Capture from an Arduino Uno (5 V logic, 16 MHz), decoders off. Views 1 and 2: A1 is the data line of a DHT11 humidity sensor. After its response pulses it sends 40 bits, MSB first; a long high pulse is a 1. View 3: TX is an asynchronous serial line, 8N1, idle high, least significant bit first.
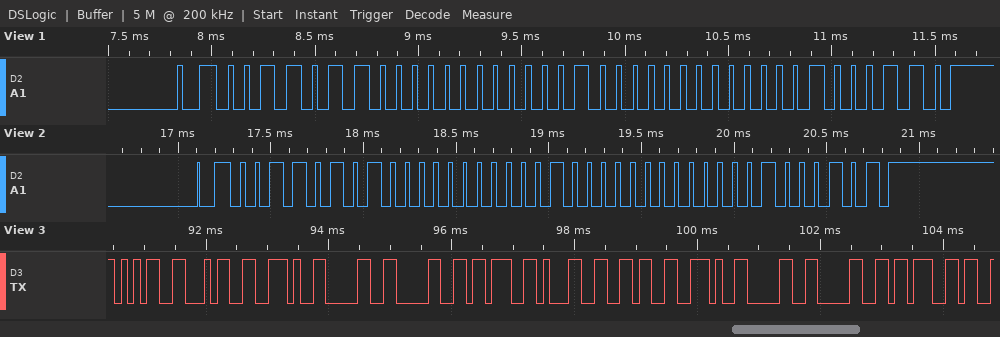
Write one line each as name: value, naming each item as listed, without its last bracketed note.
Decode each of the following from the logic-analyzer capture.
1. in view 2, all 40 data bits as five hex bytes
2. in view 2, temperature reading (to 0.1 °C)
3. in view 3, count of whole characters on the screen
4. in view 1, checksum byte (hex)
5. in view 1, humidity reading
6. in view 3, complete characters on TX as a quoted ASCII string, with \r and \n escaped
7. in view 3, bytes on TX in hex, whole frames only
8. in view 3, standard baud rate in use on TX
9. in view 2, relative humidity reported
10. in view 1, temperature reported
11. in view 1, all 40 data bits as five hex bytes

in view 2, all 40 data bits as five hex bytes: 35 00 10 00 45
in view 2, temperature reading: 16.0 °C
in view 3, count of whole characters on the screen: 12
in view 1, checksum byte: 0x46
in view 1, humidity reading: 54 %
in view 3, complete characters on TX as a quoted ASCII string, with \r and \n escaped: "54.00;16.00;"
in view 3, bytes on TX in hex, whole frames only: 35 34 2E 30 30 3B 31 36 2E 30 30 3B
in view 3, standard baud rate in use on TX: 9600 baud
in view 2, relative humidity reported: 53 %
in view 1, temperature reported: 16.0 °C
in view 1, all 40 data bits as five hex bytes: 36 00 10 00 46
